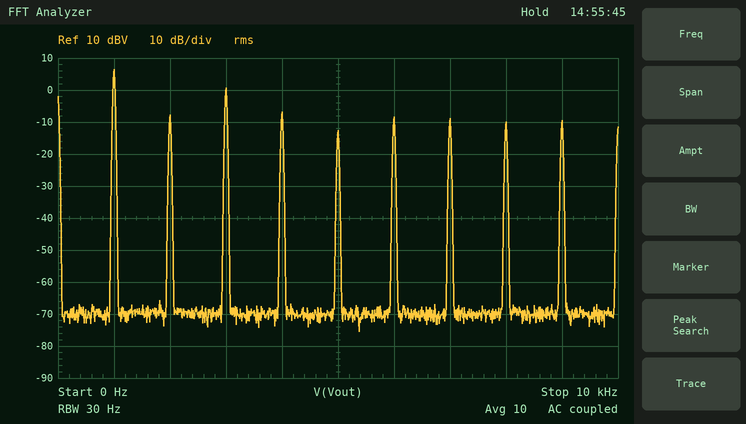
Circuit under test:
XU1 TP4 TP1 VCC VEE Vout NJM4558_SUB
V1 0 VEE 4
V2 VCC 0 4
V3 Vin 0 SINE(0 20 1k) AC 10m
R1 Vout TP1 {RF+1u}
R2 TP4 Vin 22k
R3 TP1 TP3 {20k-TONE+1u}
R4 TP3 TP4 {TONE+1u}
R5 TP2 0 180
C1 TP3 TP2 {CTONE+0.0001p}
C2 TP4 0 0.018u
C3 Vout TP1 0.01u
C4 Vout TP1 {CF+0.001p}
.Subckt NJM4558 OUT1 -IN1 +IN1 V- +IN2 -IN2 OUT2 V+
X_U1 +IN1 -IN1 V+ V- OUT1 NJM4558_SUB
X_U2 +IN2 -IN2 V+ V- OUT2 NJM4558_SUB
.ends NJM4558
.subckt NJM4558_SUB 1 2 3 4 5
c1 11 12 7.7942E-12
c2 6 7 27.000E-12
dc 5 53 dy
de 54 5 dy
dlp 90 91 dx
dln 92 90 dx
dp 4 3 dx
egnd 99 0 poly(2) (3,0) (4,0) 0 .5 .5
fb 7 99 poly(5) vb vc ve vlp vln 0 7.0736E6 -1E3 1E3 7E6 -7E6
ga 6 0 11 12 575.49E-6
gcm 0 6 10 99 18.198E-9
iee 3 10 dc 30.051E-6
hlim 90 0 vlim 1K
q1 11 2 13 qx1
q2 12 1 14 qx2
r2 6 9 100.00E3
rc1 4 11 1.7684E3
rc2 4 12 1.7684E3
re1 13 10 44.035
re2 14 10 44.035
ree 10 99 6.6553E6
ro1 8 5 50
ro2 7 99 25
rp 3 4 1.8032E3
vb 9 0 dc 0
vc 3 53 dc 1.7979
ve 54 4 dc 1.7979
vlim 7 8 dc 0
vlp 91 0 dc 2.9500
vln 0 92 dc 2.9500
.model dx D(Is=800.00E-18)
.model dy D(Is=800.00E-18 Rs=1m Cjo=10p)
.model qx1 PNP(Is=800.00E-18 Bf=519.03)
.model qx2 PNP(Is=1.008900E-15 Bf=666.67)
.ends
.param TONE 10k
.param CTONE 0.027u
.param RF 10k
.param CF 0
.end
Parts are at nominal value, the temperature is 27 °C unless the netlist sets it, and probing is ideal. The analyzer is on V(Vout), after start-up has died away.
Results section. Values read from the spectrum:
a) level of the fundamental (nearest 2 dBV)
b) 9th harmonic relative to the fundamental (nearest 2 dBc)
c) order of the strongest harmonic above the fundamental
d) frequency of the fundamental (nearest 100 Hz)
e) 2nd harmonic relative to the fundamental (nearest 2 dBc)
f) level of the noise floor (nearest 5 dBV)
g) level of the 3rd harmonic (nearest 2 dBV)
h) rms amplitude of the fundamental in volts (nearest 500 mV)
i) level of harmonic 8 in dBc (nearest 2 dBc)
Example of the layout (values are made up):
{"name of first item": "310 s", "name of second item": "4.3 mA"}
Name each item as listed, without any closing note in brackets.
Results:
{"level of the fundamental": "6 dBV", "9th harmonic relative to the fundamental": "-16 dBc", "order of the strongest harmonic above the fundamental": "3", "frequency of the fundamental": "1.0 kHz", "2nd harmonic relative to the fundamental": "-14 dBc", "level of the noise floor": "-70 dBV", "level of the 3rd harmonic": "0 dBV", "rms amplitude of the fundamental in volts": "2.0 V", "level of harmonic 8 in dBc": "-16 dBc"}
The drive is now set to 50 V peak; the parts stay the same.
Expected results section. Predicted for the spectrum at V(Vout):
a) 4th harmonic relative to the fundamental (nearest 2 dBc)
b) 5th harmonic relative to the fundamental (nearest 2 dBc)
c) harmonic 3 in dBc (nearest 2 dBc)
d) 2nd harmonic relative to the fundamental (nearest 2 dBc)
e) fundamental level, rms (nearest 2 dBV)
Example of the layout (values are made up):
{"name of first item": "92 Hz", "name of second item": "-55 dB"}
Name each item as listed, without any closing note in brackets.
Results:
{"4th harmonic relative to the fundamental": "-10 dBc", "5th harmonic relative to the fundamental": "2 dBc", "harmonic 3 in dBc": "6 dBc", "2nd harmonic relative to the fundamental": "4 dBc", "fundamental level, rms": "-4 dBV"}
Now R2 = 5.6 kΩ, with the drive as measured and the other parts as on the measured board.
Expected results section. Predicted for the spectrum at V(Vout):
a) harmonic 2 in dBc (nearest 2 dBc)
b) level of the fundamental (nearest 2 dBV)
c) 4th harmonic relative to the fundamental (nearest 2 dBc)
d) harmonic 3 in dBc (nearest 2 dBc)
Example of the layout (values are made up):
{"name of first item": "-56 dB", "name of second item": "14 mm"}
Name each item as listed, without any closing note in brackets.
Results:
{"harmonic 2 in dBc": "8 dBc", "level of the fundamental": "-8 dBV", "4th harmonic relative to the fundamental": "2 dBc", "harmonic 3 in dBc": "6 dBc"}
